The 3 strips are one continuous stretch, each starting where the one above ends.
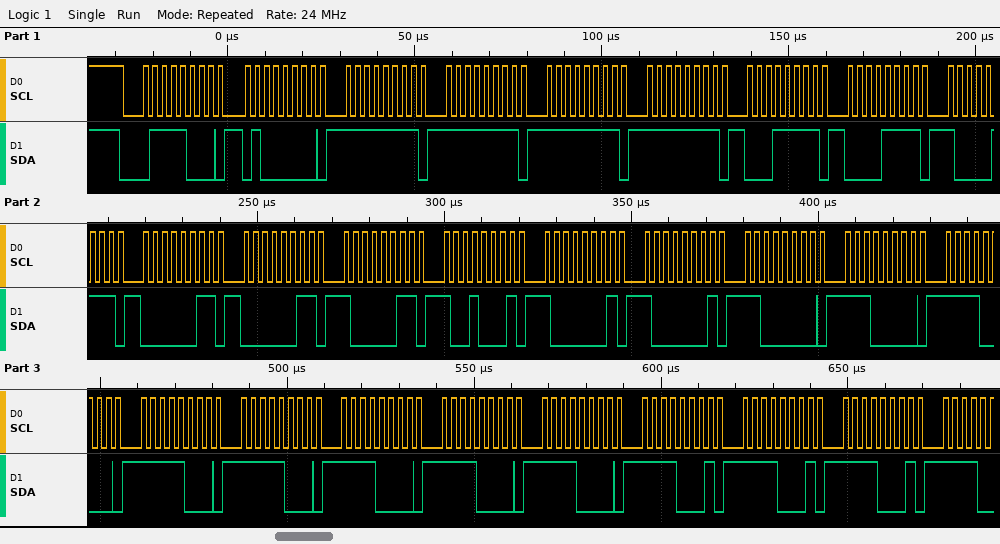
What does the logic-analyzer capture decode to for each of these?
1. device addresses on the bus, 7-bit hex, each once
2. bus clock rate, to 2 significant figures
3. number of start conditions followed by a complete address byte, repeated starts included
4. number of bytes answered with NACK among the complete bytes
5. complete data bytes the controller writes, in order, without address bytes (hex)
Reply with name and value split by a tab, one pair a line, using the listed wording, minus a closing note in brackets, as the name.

device addresses on the bus, 7-bit hex, each once	0x3C
bus clock rate, to 2 significant figures	400 kHz
number of start conditions followed by a complete address byte, repeated starts included	1
number of bytes answered with NACK among the complete bytes	0
complete data bytes the controller writes, in order, without address bytes	40 FF FF FF FF 1F 0F 87 03 03 83 91 81 81 C0 E0 F0 F8 F8 F0 F0 F0 F1 F1 F1
